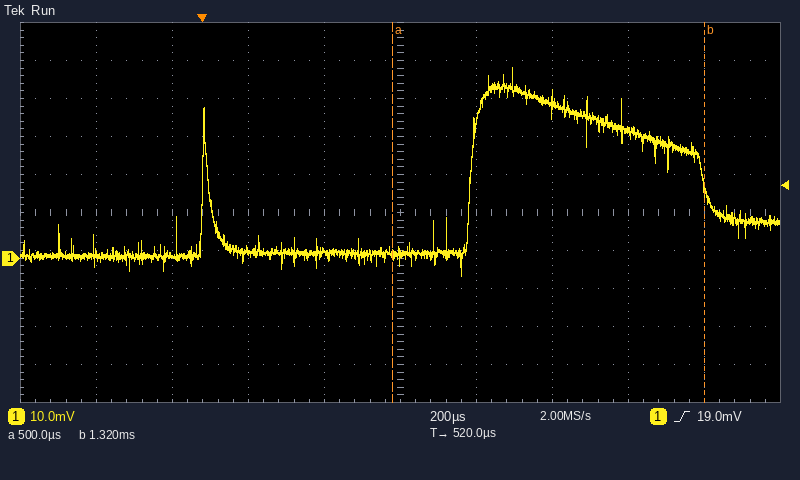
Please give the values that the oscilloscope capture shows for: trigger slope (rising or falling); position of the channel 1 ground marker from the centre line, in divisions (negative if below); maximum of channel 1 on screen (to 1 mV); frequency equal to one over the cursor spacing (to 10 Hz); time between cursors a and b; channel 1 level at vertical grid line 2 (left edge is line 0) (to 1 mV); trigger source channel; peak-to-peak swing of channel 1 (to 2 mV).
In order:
rising
-1.2 div
50 mV
1.22 kHz
820 µs
1 mV
channel 1
54 mV
